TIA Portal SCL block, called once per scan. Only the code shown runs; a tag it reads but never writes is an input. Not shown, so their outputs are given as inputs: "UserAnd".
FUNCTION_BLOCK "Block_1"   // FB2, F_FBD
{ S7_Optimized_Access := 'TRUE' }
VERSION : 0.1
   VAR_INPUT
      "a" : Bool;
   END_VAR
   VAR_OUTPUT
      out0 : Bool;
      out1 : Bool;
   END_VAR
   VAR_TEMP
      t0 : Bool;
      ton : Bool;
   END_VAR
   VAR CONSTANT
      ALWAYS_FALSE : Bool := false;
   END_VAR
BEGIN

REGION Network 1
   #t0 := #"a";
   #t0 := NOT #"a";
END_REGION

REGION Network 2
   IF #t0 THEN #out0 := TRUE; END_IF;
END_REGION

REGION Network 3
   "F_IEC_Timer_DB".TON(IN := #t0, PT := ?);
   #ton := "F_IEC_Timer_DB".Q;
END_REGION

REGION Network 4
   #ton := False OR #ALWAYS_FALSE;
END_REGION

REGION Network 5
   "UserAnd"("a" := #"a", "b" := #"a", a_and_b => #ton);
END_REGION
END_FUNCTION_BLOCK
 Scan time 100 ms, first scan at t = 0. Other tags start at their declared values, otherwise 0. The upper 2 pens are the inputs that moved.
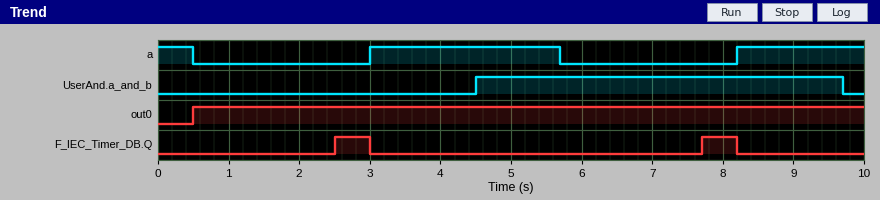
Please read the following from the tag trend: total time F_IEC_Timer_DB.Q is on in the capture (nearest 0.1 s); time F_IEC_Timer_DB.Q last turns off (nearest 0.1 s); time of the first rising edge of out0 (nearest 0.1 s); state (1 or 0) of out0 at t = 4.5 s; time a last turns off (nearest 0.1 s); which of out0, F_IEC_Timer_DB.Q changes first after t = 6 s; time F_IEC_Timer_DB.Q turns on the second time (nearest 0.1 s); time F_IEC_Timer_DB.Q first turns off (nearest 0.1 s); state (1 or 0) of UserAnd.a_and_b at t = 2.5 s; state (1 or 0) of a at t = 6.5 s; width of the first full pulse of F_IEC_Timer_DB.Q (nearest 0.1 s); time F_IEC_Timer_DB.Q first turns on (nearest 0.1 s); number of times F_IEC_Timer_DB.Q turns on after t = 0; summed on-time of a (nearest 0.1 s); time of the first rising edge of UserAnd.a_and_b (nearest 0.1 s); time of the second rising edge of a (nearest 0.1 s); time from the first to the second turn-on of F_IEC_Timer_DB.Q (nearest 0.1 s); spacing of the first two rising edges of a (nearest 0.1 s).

1.0 s
8.2 s
0.5 s
1
5.7 s
F_IEC_Timer_DB.Q
7.7 s
3.0 s
0
0
0.5 s
2.5 s
2
5.0 s
4.5 s
8.2 s
5.2 s
5.2 s
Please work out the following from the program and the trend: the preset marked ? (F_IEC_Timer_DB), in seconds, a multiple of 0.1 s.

2.0 s
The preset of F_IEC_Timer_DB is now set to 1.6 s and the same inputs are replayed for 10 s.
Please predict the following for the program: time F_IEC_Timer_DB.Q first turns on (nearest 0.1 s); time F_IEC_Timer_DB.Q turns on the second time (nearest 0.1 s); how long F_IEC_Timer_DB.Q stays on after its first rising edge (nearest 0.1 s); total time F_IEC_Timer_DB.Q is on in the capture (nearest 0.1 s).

2.1 s
7.3 s
0.9 s
1.8 s
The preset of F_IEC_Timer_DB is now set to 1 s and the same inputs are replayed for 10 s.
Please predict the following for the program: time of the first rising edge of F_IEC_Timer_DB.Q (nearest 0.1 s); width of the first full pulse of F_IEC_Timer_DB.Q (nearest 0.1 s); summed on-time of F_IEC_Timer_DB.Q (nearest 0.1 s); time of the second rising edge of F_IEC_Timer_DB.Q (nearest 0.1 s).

1.5 s
1.5 s
3.0 s
6.7 s
